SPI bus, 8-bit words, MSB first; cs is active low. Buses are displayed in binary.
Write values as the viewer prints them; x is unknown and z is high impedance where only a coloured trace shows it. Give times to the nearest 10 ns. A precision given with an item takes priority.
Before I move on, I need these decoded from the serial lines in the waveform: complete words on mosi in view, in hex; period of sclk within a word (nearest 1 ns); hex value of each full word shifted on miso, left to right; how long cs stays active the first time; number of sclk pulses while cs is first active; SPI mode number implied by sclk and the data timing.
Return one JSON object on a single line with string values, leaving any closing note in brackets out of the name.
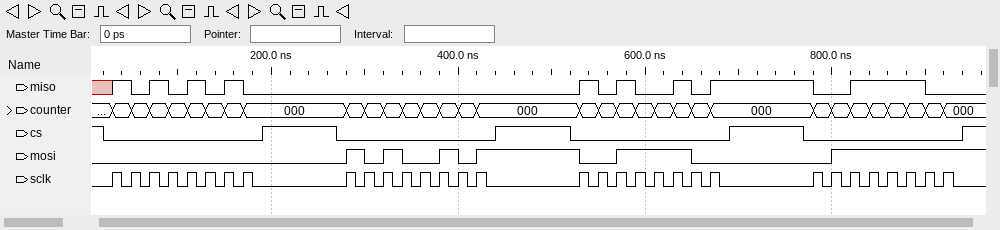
{"complete words on mosi in view, in hex": "00, A5, 3C, 7F", "period of sclk within a word": "20 ns", "hex value of each full word shifted on miso, left to right": "AA, 00, A5, 3C", "how long cs stays active the first time": "170 ns", "number of sclk pulses while cs is first active": "8", "SPI mode number implied by sclk and the data timing": "1"}
